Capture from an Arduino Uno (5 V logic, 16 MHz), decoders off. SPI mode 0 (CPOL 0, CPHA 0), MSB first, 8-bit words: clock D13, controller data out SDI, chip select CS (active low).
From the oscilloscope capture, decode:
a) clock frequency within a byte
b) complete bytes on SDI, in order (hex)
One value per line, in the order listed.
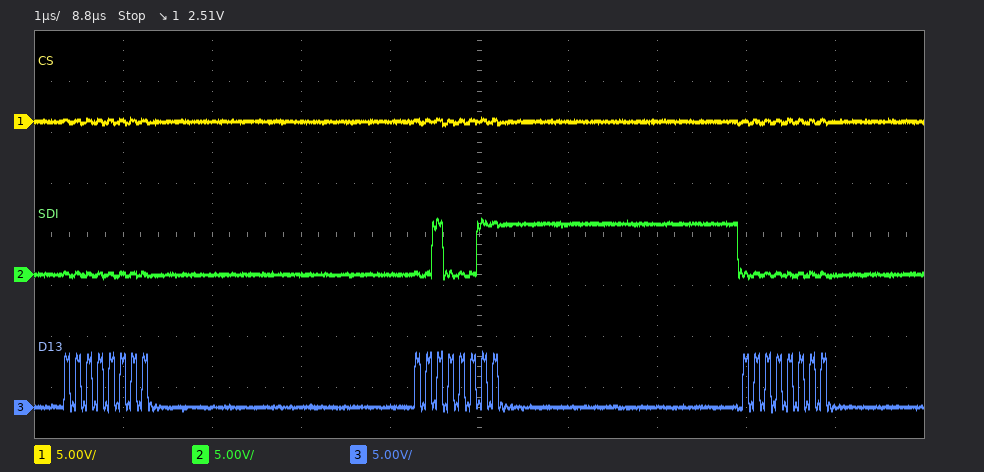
8 MHz
00 23 00
